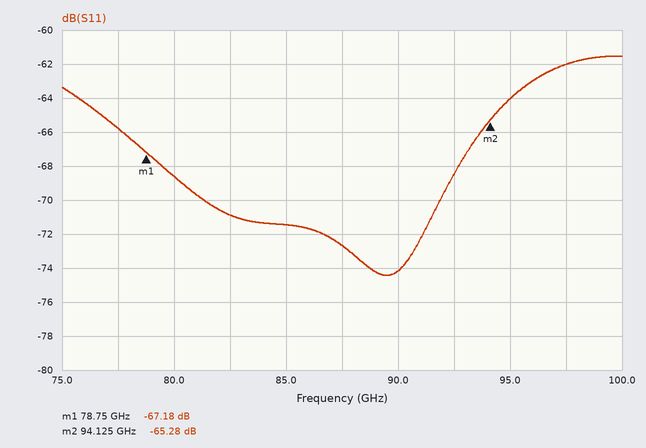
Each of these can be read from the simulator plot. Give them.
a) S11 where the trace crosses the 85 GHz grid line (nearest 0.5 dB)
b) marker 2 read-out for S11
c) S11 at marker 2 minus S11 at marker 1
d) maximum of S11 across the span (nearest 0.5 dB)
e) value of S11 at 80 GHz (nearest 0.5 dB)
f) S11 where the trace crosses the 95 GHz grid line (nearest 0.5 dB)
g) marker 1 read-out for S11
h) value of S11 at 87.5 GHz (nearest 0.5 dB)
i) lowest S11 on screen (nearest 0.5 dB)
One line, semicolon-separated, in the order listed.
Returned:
-71.5 dB; -65.28 dB; 1.90 dB; -61.5 dB; -68.5 dB; -64.0 dB; -67.18 dB; -72.5 dB; -74.5 dB
